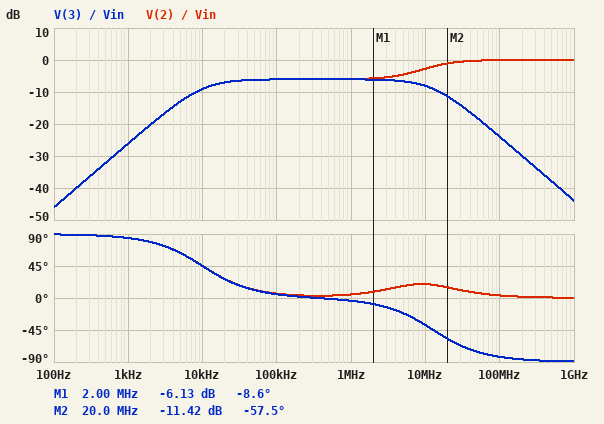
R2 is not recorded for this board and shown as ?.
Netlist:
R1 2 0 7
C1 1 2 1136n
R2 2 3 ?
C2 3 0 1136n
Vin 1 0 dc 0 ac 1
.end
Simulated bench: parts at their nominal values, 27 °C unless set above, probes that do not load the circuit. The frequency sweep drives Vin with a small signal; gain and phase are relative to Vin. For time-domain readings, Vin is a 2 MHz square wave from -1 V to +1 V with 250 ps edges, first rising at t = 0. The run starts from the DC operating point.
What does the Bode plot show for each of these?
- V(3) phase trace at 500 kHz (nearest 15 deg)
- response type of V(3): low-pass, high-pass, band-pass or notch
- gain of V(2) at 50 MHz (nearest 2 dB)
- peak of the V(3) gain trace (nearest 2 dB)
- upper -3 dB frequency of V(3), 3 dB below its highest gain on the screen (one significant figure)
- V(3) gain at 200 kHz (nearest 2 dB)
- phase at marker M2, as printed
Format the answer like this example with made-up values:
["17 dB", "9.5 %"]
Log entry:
["0 deg", "band-pass", "0 dB", "-6 dB", "10 MHz", "-6 dB", "-57.5 deg"]
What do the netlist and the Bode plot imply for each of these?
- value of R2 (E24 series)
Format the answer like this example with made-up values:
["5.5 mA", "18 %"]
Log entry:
["0.022 Ω"]
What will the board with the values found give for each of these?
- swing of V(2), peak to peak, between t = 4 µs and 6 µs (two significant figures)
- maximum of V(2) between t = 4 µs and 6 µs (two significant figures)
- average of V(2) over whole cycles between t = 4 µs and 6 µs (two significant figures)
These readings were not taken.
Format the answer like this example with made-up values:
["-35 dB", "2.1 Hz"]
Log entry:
["3.0 V", "1.9 V", "360 mV"]
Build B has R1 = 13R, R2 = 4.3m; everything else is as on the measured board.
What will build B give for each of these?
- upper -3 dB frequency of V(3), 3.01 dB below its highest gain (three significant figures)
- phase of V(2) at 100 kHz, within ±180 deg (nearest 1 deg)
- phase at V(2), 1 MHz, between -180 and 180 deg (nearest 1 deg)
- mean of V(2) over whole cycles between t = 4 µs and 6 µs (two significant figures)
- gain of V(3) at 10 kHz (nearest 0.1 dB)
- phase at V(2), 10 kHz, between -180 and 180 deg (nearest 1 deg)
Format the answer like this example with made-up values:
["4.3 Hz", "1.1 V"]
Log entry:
["65.2 MHz", "3 deg", "1 deg", "420 mV", "-7.1 dB", "28 deg"]
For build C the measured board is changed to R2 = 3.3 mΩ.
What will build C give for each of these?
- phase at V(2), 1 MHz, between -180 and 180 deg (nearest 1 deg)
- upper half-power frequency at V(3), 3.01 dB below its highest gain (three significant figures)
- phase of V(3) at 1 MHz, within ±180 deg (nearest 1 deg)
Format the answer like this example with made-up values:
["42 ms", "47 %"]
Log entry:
["1 deg", "84.9 MHz", "0 deg"]
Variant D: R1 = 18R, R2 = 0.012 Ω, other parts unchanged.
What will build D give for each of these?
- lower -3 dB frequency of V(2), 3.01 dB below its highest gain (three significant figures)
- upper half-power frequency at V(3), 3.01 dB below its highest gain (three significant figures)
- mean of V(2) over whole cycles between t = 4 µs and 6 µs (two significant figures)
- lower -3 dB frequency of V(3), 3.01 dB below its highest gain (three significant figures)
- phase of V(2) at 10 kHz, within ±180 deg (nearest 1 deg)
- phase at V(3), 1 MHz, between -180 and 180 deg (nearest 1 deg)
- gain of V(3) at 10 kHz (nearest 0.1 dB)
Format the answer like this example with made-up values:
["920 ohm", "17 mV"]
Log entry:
["16.5 MHz", "23.4 MHz", "440 mV", "3.89 kHz", "21 deg", "-2 deg", "-6.6 dB"]
